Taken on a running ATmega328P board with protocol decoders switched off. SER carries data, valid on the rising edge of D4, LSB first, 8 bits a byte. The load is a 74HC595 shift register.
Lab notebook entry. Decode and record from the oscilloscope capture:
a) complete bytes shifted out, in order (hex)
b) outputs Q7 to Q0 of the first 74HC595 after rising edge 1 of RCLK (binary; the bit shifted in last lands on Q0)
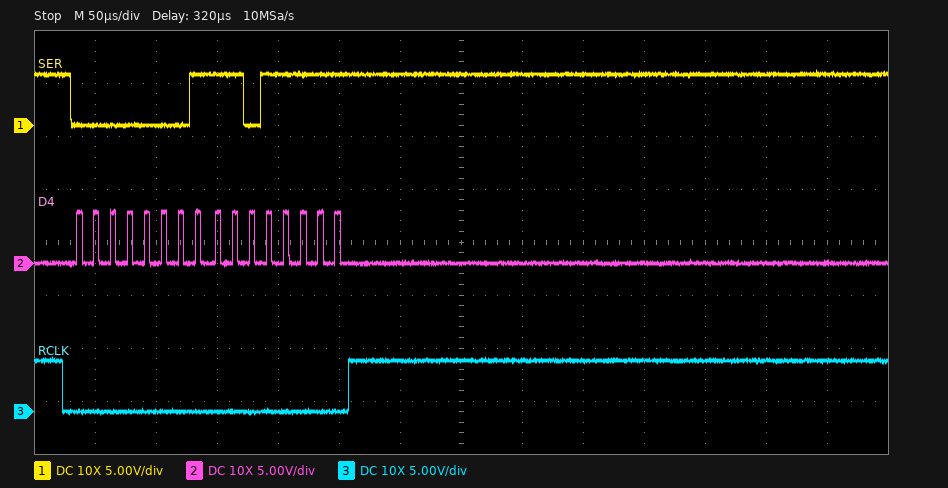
0x80 0xFB
11011111
